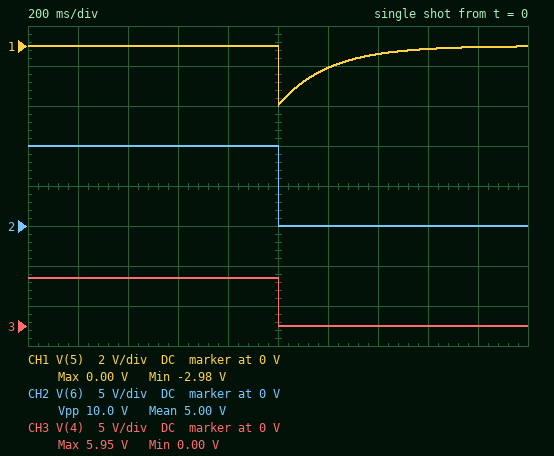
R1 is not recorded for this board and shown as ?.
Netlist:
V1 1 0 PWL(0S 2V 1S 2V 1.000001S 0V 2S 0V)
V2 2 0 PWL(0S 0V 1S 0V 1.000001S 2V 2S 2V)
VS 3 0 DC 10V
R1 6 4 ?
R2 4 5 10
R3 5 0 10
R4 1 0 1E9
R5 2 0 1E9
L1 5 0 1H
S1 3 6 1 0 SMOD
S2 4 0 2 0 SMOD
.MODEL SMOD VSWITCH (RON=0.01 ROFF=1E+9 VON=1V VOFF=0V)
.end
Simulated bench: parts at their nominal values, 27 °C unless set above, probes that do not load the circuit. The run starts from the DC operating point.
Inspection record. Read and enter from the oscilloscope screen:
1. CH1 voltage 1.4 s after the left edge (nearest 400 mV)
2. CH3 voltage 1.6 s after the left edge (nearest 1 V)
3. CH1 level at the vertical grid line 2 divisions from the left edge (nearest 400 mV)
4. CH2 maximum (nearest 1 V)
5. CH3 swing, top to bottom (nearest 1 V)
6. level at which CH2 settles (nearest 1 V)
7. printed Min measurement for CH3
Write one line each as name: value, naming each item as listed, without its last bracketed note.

CH1 voltage 1.4 s after the left edge: -400 mV
CH3 voltage 1.6 s after the left edge: 0 V
CH1 level at the vertical grid line 2 divisions from the left edge: 0 V
CH2 maximum: 10 V
CH3 swing, top to bottom: 6 V
level at which CH2 settles: 0 V
printed Min measurement for CH3: 0.00 V
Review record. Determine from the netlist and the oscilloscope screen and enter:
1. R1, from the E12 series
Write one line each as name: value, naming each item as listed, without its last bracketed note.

R1, from the E12 series: 6.8 Ω
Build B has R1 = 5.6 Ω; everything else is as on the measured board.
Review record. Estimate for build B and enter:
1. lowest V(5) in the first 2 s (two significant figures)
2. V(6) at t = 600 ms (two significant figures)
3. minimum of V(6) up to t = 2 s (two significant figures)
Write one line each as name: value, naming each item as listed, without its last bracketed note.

lowest V(5) in the first 2 s: -3.2 V
V(6) at t = 600 ms: 10 V
minimum of V(6) up to t = 2 s: -3.2 mV
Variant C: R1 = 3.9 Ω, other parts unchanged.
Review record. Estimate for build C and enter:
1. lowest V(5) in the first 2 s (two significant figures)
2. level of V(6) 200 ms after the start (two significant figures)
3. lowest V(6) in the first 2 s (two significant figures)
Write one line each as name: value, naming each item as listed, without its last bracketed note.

lowest V(5) in the first 2 s: -3.6 V
level of V(6) 200 ms after the start: 10 V
lowest V(6) in the first 2 s: -3.6 mV
